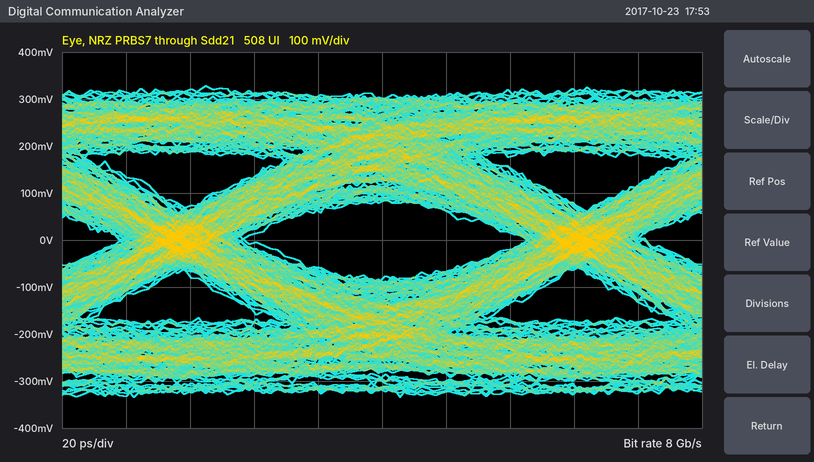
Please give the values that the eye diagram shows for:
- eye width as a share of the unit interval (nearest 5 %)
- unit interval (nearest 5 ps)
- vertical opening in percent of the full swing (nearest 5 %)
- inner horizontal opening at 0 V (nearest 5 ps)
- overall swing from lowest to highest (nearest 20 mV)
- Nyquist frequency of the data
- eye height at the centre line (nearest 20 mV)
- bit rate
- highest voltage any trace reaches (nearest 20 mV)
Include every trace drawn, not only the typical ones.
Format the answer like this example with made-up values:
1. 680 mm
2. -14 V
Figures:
1. 70 %
2. 125 ps
3. 25 %
4. 90 ps
5. 660 mV
6. 4 GHz
7. 160 mV
8. 8 Gb/s
9. 320 mV
